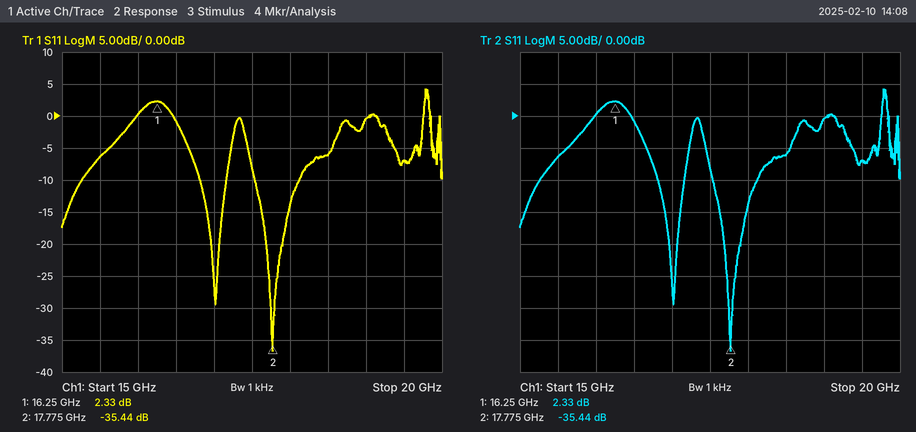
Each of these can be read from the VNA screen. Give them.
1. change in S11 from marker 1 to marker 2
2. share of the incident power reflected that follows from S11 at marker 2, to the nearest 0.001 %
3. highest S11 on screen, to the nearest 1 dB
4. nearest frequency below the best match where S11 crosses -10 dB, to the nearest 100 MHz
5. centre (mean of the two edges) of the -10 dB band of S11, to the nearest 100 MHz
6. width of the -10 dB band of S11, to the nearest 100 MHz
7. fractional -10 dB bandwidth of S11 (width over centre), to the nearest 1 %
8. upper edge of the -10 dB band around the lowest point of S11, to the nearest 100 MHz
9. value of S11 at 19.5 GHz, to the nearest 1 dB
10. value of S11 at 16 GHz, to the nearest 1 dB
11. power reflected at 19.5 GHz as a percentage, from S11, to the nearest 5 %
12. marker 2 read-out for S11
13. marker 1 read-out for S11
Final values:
-37.77 dB
0.029 %
4 dB
17.5 GHz
17.8 GHz
600 MHz
3 %
18.1 GHz
-7 dB
0 dB
20 %
-35.44 dB
2.33 dB
